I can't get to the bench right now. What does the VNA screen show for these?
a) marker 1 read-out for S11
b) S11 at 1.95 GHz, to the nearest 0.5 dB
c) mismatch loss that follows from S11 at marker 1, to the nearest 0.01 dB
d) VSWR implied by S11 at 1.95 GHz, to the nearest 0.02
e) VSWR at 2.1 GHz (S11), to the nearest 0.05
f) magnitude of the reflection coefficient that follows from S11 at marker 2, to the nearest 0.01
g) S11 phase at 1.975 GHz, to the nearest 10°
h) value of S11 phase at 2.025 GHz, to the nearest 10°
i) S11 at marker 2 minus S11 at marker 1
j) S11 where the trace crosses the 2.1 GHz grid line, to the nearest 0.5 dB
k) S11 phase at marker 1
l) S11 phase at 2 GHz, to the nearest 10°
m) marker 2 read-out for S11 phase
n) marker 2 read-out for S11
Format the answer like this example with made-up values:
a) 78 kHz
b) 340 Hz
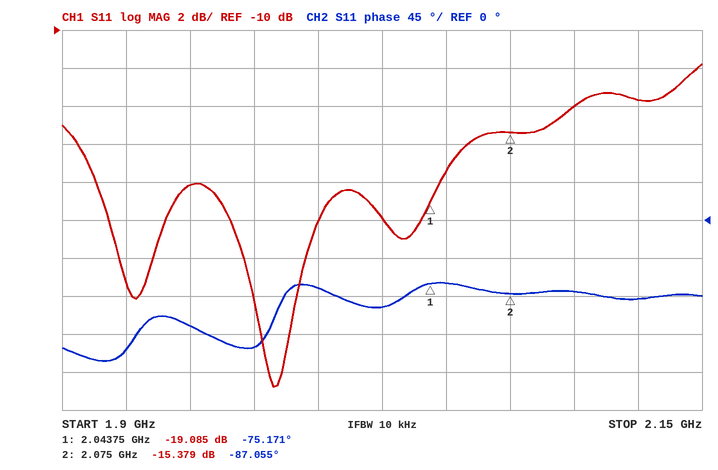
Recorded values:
a) -19.085 dB
b) -18.0 dB
c) 0.05 dB
d) 1.28
e) 1.50
f) 0.17
g) -150°
h) -100°
i) 3.706 dB
j) -14.0 dB
k) -75.171°
l) -80°
m) -87.055°
n) -15.379 dB
